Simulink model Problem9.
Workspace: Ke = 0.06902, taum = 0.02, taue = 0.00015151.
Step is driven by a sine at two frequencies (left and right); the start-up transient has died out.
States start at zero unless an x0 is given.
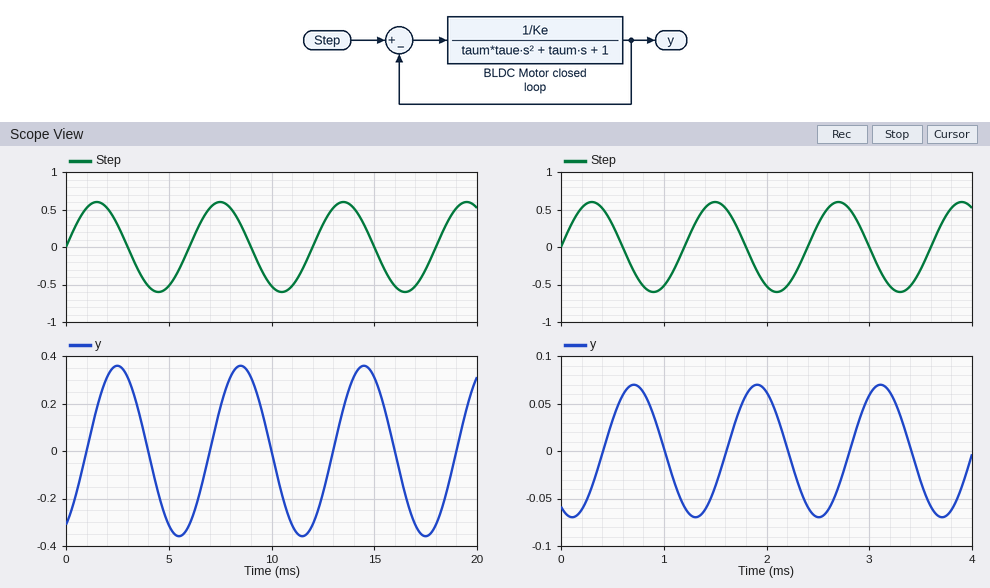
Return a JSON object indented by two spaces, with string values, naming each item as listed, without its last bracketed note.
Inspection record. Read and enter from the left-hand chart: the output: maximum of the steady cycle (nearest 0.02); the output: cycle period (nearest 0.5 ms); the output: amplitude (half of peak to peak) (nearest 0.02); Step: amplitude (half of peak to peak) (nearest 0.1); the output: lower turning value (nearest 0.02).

{
  "the output: maximum of the steady cycle": "0.36",
  "the output: cycle period": "6.0 ms",
  "the output: amplitude (half of peak to peak)": "0.36",
  "Step: amplitude (half of peak to peak)": "0.6",
  "the output: lower turning value": "-0.36"
}
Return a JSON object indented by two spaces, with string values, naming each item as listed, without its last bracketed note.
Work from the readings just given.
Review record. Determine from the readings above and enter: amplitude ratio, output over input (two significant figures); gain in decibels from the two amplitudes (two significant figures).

{
  "amplitude ratio, output over input": "0.60",
  "gain in decibels from the two amplitudes": "-4.4 dB"
}
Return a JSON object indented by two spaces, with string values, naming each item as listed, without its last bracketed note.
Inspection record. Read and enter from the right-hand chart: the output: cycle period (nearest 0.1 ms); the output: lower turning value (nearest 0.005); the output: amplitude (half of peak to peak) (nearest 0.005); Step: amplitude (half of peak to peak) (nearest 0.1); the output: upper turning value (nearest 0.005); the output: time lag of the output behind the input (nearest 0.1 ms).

{
  "the output: cycle period": "1.2 ms",
  "the output: lower turning value": "-0.070",
  "the output: amplitude (half of peak to peak)": "0.070",
  "Step: amplitude (half of peak to peak)": "0.6",
  "the output: upper turning value": "0.070",
  "the output: time lag of the output behind the input": "0.4 ms"
}
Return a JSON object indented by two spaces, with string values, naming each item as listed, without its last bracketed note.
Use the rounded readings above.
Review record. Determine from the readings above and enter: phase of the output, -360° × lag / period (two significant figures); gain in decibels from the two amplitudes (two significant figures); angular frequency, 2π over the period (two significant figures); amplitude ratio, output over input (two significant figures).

{
  "phase of the output, -360° × lag / period": "-120°",
  "gain in decibels from the two amplitudes": "-19 dB",
  "angular frequency, 2π over the period": "5.2 rad/ms",
  "amplitude ratio, output over input": "0.12"
}
